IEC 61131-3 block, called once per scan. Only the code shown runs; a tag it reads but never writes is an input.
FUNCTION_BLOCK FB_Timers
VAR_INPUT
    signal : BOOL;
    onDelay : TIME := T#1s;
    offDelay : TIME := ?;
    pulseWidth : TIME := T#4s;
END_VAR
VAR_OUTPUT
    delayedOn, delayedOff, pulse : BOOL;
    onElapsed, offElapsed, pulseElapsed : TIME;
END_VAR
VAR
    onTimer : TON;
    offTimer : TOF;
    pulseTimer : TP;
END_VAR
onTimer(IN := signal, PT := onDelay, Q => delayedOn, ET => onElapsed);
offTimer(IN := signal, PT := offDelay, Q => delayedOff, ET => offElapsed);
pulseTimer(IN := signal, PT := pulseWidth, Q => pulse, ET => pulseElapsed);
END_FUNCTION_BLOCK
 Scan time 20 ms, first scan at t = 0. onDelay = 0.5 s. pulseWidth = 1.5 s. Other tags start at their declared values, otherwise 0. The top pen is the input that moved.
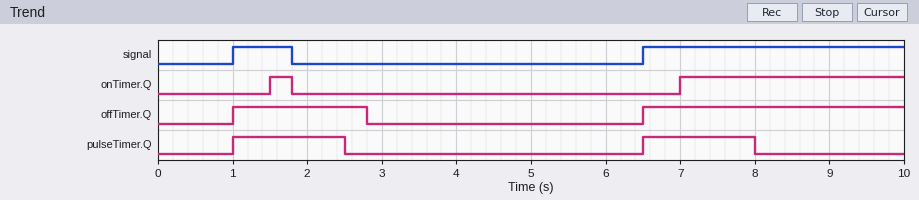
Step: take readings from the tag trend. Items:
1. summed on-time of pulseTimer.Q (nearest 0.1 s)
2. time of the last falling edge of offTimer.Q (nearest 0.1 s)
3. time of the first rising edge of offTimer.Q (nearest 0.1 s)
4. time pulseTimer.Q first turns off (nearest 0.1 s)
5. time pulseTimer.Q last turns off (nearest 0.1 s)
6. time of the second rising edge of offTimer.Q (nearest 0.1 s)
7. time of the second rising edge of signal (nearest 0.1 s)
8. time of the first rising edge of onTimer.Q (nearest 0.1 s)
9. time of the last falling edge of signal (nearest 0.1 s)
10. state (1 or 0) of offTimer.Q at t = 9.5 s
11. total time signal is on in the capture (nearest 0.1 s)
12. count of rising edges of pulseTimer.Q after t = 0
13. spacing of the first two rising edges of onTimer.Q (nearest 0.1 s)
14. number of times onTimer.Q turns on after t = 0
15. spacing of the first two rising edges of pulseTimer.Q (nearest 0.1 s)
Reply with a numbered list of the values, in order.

1. 3.0 s
2. 2.8 s
3. 1.0 s
4. 2.5 s
5. 8.0 s
6. 6.5 s
7. 6.5 s
8. 1.5 s
9. 1.8 s
10. 1
11. 4.3 s
12. 2
13. 5.5 s
14. 2
15. 5.5 s
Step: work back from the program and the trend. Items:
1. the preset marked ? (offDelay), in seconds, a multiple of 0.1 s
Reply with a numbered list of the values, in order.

1. 1.0 s
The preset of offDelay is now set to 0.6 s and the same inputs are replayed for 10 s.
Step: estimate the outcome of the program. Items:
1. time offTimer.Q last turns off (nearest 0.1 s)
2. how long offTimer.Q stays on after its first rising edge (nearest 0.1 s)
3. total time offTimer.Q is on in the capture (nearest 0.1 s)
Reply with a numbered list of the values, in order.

1. 2.4 s
2. 1.4 s
3. 4.9 s
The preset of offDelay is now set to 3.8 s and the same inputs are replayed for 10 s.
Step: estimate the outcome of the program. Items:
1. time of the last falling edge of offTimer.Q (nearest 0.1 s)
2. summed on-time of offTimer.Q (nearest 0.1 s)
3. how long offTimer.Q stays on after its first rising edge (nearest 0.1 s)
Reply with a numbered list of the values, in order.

1. 5.6 s
2. 8.1 s
3. 4.6 s
